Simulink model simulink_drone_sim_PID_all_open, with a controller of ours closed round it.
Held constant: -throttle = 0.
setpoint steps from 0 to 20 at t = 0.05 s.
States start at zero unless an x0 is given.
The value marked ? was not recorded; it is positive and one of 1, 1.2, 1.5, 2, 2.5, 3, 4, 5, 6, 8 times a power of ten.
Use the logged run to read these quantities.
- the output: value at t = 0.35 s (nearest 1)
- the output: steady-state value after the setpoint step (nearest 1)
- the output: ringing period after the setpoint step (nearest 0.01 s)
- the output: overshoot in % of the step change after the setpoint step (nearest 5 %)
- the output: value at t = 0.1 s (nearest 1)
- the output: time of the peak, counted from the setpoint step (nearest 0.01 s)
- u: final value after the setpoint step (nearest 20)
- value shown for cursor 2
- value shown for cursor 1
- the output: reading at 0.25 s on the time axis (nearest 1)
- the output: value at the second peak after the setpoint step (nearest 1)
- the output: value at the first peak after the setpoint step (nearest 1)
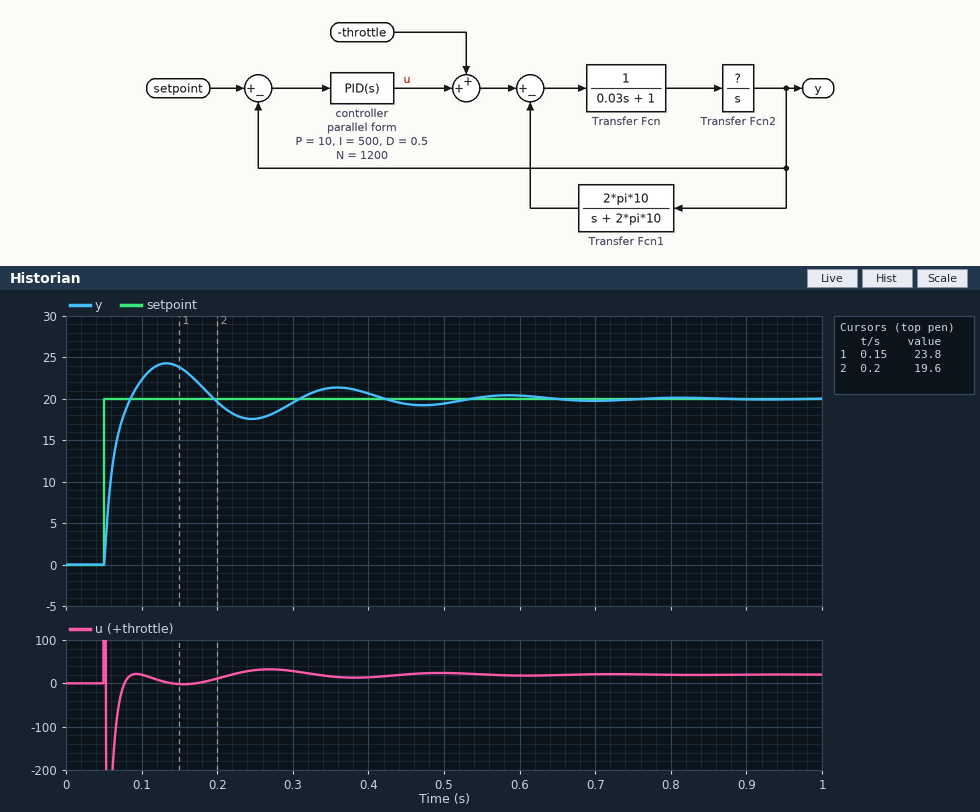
21
20
0.23 s
20 %
22
0.08 s
20
19.6
23.8
18
21
24
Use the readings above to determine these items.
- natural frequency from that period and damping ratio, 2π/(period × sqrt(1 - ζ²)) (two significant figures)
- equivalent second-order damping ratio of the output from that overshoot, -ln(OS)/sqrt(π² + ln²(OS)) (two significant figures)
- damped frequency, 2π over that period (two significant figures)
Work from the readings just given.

31 rad/s
0.46
27 rad/s
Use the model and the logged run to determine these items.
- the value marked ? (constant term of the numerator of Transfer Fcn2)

5
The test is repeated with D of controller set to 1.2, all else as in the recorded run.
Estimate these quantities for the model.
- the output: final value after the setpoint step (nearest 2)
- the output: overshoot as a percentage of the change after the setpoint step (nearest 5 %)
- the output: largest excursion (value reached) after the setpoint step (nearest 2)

20
10 %
22
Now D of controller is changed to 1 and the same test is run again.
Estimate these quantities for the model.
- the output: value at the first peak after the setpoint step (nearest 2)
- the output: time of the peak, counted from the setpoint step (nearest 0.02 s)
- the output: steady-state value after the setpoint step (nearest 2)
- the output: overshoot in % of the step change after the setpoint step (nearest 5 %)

22
0.12 s
20
10 %
